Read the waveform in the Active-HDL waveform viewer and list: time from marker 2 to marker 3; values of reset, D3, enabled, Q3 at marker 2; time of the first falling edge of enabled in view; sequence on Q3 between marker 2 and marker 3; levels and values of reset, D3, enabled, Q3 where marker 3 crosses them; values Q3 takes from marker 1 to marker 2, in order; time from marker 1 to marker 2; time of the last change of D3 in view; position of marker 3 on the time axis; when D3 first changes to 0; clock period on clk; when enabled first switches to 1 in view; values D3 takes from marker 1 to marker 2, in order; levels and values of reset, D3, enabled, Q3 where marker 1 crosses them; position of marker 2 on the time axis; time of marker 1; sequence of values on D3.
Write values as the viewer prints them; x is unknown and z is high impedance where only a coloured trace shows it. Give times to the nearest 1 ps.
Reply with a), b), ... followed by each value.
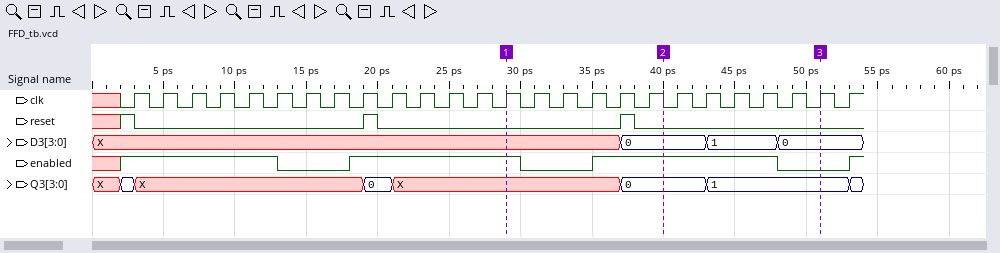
a) 11 ps
b) reset=0, D3=0, enabled=1, Q3=0
c) 13 ps
d) 0, 1
e) reset=0, D3=0, enabled=0, Q3=1
f) X, 0
g) 11 ps
h) 48 ps
i) 51 ps
j) 37 ps
k) 2 ps
l) 2 ps
m) X, 0
n) reset=0, D3=X, enabled=1, Q3=X
o) 40 ps
p) 29 ps
q) X, 0, 1, 0
